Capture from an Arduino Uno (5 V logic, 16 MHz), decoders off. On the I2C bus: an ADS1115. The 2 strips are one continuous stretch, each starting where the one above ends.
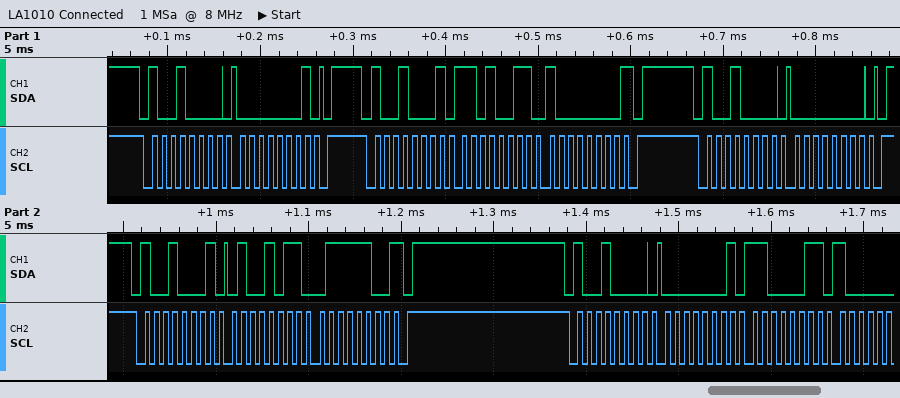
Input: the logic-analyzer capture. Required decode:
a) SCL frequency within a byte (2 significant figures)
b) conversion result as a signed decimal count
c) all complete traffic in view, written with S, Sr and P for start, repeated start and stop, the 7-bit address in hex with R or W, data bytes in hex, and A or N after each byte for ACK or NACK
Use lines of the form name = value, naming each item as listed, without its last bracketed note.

SCL frequency within a byte = 100 kHz
conversion result as a signed decimal count = 19324
all complete traffic in view, written with S, Sr and P for start, repeated start and stop, the 7-bit address in hex with R or W, data bytes in hex, and A or N after each byte for ACK or NACK = S 48W A 01 A P S 48R A D3 A 80 N P S 48W A 00 A P S 48R A 4B A 7C N P S 48W A 01 A C3 A
